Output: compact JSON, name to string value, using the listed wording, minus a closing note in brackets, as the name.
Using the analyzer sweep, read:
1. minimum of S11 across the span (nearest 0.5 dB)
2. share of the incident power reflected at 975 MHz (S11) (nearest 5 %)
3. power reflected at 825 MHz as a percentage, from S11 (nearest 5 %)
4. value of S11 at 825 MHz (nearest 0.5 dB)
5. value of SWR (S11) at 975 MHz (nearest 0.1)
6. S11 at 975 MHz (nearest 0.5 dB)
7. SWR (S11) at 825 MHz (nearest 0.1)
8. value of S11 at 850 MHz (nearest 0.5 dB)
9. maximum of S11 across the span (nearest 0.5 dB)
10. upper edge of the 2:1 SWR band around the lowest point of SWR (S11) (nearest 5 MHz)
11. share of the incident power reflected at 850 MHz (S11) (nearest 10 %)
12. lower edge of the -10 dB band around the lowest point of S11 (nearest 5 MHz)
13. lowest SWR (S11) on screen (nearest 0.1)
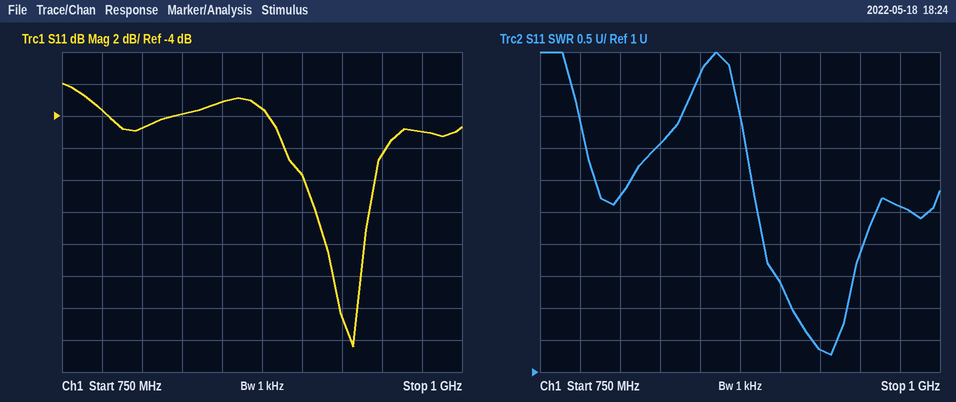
{"minimum of S11 across the span": "-18.5 dB", "share of the incident power reflected at 975 MHz (S11)": "30 %", "power reflected at 825 MHz as a percentage, from S11": "40 %", "value of S11 at 825 MHz": "-4.0 dB", "value of SWR (S11) at 975 MHz": "3.6", "S11 at 975 MHz": "-5.0 dB", "SWR (S11) at 825 MHz": "4.6", "value of S11 at 850 MHz": "-3.0 dB", "maximum of S11 across the span": "-2.0 dB", "upper edge of the 2:1 SWR band around the lowest point of SWR (S11)": "940 MHz", "share of the incident power reflected at 850 MHz (S11)": "50 %", "lower edge of the -10 dB band around the lowest point of S11": "910 MHz", "lowest SWR (S11) on screen": "1.3"}
